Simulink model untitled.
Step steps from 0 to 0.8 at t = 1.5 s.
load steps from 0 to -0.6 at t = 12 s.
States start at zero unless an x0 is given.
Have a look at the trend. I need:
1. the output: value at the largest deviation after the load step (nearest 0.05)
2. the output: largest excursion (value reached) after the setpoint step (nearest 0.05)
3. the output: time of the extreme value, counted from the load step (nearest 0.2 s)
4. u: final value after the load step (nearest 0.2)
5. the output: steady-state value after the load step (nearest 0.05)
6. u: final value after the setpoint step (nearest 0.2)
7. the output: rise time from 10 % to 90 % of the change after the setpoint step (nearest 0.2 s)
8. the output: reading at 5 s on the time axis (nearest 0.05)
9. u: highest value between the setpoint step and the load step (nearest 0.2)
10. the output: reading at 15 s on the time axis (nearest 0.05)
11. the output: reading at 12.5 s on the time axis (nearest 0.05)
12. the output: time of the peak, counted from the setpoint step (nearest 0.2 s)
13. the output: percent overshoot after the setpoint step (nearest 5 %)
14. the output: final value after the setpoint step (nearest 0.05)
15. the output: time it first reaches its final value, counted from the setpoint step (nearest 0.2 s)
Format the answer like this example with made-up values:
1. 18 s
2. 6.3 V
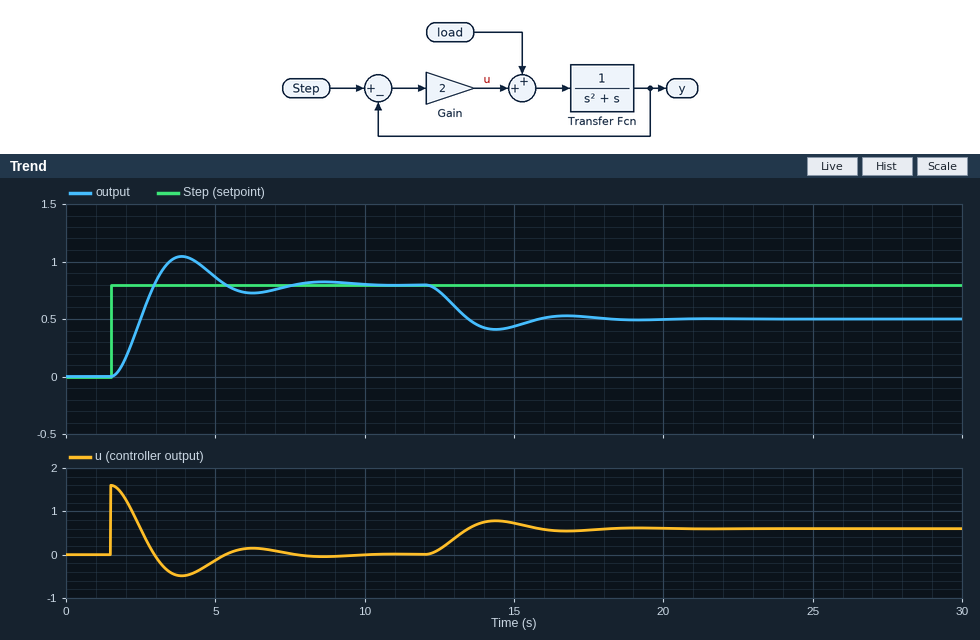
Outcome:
1. 0.40
2. 1.05
3. 2.4 s
4. 0.6
5. 0.50
6. 0.0
7. 1.0 s
8. 0.85
9. 1.6
10. 0.45
11. 0.75
12. 2.4 s
13. 30 %
14. 0.80
15. 1.4 s
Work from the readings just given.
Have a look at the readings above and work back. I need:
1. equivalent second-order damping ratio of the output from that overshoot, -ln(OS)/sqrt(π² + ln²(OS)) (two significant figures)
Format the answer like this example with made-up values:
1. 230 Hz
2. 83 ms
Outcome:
1. 0.36
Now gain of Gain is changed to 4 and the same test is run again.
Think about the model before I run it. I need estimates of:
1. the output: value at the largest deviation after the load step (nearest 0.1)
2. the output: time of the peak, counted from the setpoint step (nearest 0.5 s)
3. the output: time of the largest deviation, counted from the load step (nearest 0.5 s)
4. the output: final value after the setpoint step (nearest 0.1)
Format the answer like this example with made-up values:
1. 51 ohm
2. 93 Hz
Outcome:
1. 0.6
2. 1.5 s
3. 1.5 s
4. 0.8
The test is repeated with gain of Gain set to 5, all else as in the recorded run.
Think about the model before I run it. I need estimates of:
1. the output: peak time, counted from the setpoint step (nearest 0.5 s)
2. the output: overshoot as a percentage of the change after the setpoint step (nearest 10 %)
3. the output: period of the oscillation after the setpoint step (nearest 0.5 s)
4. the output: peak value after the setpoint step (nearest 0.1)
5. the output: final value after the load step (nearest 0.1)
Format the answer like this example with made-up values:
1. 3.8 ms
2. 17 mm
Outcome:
1. 1.5 s
2. 50 %
3. 3.0 s
4. 1.2
5. 0.7
